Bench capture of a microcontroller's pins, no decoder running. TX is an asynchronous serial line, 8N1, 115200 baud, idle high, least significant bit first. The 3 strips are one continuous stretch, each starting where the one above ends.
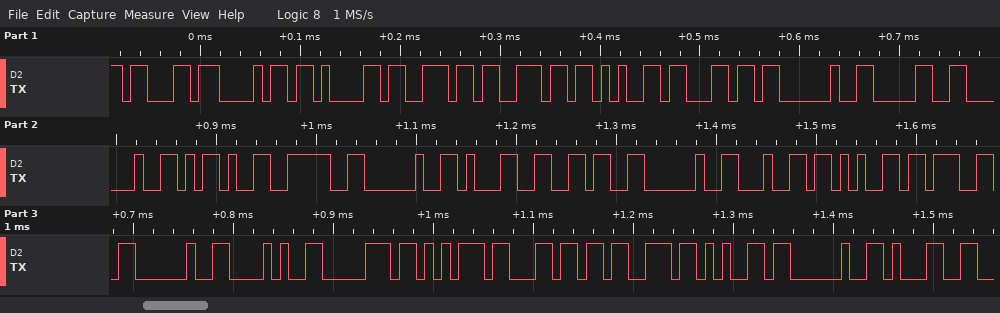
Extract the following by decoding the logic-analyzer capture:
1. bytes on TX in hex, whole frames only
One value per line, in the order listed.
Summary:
63 68 61 6E 6E 65 6C 20 30 20 2D 3E 20 31 36 20 64 65 67 20 28 70 75 6C 73 65 20 31
